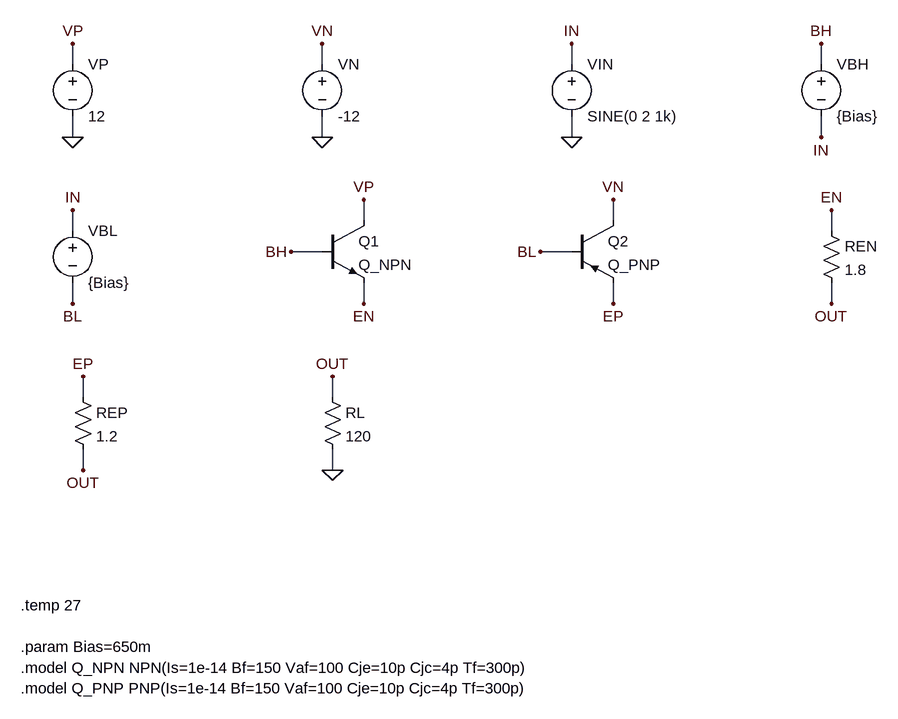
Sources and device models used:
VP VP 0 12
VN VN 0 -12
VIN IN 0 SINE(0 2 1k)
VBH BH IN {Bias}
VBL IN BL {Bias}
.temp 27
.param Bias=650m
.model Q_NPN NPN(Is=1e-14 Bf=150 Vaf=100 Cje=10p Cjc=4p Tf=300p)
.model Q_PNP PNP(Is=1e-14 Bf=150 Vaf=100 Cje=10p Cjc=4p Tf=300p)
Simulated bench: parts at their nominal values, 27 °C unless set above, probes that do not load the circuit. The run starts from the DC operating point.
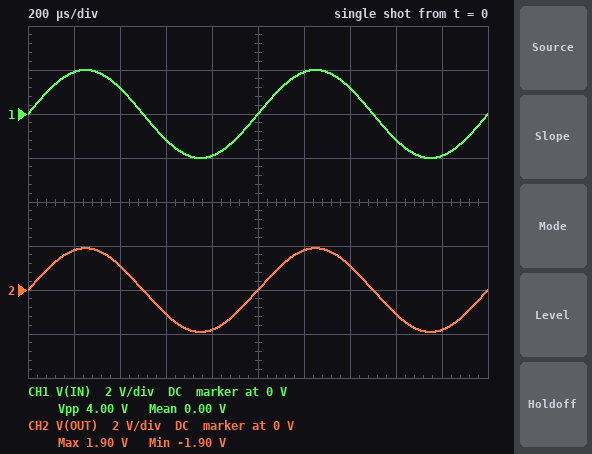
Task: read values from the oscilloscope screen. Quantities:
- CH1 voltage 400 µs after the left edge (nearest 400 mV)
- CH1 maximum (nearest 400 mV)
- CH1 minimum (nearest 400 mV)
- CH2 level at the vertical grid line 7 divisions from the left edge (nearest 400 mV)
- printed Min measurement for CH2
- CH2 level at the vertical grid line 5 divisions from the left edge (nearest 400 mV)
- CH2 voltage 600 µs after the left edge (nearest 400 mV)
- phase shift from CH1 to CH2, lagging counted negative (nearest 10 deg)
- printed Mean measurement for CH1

1.2 V
2.0 V
-2.0 V
1.2 V
-1.90 V
0 V
-1.2 V
0 deg
0.00 V
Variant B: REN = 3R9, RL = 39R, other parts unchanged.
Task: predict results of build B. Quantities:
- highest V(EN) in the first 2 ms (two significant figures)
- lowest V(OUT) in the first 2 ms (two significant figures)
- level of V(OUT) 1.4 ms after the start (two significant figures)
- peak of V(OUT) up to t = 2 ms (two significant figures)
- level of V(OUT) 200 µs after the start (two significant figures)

1.9 V
-1.8 V
990 mV
1.7 V
1.6 V
